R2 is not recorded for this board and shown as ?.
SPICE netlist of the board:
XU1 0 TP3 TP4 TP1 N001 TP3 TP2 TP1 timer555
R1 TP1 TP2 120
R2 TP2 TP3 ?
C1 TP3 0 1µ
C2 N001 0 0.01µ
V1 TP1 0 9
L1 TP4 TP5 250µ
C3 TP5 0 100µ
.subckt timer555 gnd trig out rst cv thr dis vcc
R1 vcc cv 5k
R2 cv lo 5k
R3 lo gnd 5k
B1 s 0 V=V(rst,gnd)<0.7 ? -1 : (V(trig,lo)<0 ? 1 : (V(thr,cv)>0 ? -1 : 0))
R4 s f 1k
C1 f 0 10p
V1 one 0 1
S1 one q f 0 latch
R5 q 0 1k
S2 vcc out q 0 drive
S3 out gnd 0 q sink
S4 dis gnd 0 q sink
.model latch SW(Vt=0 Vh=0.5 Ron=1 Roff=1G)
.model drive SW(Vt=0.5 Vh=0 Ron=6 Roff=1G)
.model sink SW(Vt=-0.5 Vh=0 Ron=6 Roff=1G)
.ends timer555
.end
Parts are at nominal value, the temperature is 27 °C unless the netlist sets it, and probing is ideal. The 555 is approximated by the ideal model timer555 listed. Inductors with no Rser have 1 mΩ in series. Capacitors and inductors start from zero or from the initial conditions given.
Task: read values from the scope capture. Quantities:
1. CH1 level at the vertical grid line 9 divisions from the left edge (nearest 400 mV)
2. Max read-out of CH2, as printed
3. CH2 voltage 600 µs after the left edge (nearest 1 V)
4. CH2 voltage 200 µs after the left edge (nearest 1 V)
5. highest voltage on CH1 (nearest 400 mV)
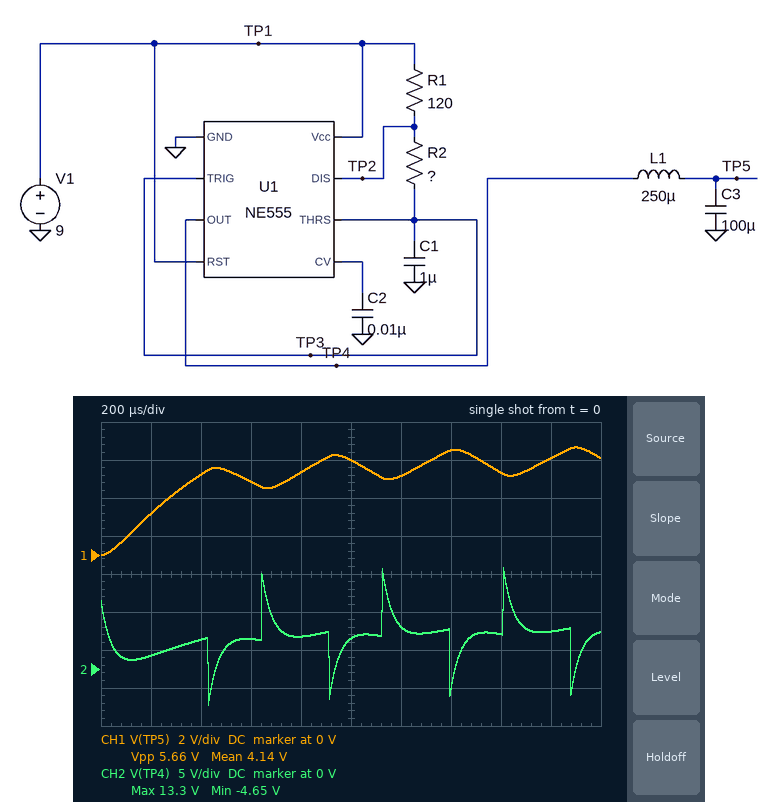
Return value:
5.2 V
13.3 V
4 V
2 V
5.6 V
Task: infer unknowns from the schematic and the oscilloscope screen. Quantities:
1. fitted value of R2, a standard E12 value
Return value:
270 Ω
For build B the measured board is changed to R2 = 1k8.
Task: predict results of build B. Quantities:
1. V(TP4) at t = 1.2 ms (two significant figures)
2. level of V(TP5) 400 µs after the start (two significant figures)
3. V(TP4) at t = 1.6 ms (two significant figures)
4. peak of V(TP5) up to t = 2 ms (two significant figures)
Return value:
7.8 V
4.2 V
8.4 V
8.7 V
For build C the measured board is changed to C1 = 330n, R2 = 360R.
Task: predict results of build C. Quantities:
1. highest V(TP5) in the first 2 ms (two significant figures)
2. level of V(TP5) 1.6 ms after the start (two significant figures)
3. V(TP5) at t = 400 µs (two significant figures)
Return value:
4.9 V
4.8 V
3.0 V
